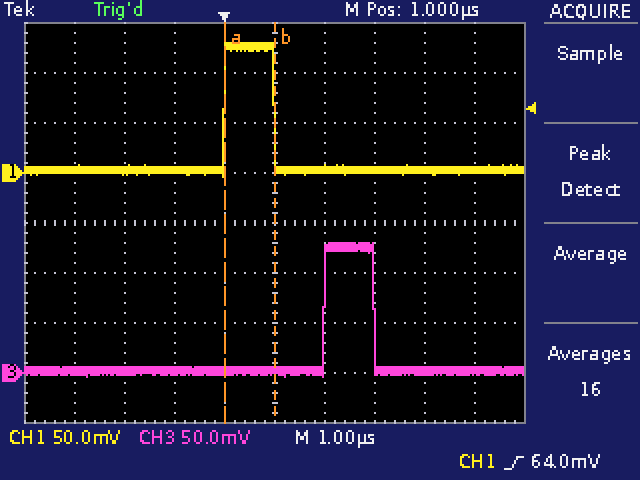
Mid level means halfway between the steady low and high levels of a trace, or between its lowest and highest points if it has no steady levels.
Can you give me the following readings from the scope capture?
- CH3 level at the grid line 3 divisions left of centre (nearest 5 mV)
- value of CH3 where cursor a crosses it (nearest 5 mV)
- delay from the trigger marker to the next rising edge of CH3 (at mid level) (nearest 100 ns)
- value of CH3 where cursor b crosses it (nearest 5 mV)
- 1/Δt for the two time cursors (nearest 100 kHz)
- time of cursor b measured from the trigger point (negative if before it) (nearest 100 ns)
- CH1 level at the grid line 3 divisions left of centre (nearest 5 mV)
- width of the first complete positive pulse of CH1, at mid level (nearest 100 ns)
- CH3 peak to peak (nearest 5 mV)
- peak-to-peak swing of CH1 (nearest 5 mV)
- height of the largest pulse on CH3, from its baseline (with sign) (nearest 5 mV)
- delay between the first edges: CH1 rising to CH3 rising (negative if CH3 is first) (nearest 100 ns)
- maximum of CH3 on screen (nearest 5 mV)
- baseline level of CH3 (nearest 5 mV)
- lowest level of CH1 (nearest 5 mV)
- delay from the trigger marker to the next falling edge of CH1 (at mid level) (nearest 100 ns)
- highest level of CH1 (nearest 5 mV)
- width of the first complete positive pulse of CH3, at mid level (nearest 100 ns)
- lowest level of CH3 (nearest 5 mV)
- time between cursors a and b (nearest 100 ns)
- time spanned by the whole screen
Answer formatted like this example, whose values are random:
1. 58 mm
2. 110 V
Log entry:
1. 0 mV
2. 0 mV
3. 2.0 µs
4. 0 mV
5. 1.0 MHz
6. +1.0 µs
7. 0 mV
8. 1.0 µs
9. 135 mV
10. 135 mV
11. +130 mV
12. +2.0 µs
13. 130 mV
14. 0 mV
15. -5 mV
16. 1.0 µs
17. 130 mV
18. 1.0 µs
19. -5 mV
20. 1.0 µs
21. 10 µs
